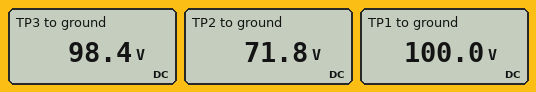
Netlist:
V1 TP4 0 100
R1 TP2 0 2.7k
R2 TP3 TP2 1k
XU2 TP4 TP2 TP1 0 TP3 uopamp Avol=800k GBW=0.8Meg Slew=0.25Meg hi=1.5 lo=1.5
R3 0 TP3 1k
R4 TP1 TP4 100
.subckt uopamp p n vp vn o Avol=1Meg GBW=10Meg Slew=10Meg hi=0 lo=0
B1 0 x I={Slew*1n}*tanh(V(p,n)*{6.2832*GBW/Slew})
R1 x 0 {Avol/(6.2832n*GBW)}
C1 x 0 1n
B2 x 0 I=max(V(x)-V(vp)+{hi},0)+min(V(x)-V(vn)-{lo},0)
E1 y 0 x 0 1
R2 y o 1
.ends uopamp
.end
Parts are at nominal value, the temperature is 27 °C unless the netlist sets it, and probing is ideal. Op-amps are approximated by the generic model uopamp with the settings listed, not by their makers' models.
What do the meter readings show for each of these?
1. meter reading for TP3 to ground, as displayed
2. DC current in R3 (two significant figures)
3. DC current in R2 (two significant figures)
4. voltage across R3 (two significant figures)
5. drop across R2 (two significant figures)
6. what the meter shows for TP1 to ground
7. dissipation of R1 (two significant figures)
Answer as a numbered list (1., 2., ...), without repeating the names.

1. 98.4 V
2. 98 mA
3. 27 mA
4. 98 V
5. 27 V
6. 100.0 V
7. 1.9 W
